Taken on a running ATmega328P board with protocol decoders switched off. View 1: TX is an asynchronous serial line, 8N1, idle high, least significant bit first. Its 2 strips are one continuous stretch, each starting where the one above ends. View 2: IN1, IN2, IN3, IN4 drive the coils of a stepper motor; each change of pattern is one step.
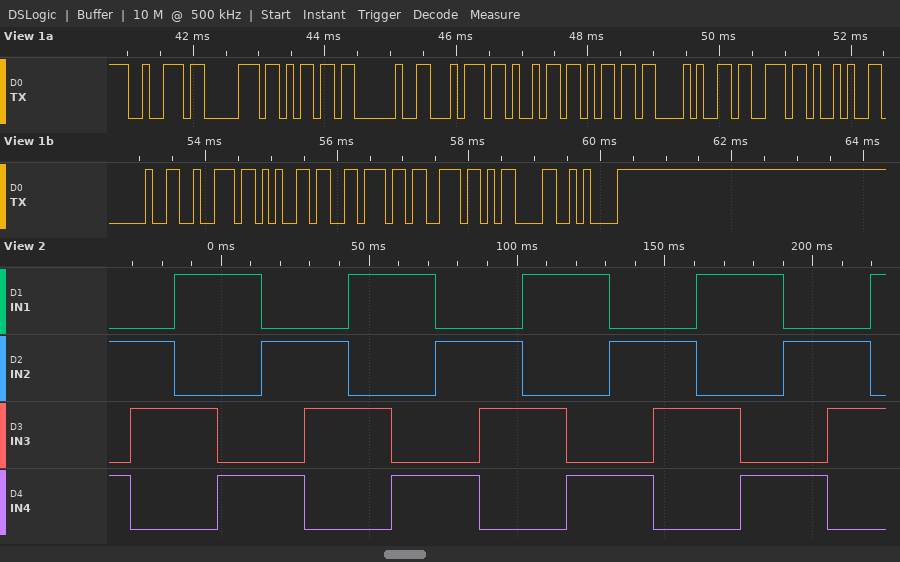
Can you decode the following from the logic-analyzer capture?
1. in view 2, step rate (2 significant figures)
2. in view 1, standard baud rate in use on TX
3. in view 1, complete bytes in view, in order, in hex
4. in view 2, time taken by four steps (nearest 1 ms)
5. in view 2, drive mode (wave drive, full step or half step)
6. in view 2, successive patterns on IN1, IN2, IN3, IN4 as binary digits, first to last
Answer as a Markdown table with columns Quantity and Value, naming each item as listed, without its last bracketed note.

| Quantity | Value |
|---|---|
| in view 2, step rate | 68 steps/s |
| in view 1, standard baud rate in use on TX | 9600 baud |
| in view 1, complete bytes in view, in order, in hex | 72 70 6D 20 74 69 6D 28 73 29 20 72 65 76 73 0D 0A |
| in view 2, time taken by four steps | 59 ms |
| in view 2, drive mode | full step |
| in view 2, successive patterns on IN1, IN2, IN3, IN4 as binary digits, first to last | 0101 0110 1010 1001 0101 0110 1010 1001 0101 0110 1010 1001 0101 0110 1010 1001 0101 0110 1010 |
